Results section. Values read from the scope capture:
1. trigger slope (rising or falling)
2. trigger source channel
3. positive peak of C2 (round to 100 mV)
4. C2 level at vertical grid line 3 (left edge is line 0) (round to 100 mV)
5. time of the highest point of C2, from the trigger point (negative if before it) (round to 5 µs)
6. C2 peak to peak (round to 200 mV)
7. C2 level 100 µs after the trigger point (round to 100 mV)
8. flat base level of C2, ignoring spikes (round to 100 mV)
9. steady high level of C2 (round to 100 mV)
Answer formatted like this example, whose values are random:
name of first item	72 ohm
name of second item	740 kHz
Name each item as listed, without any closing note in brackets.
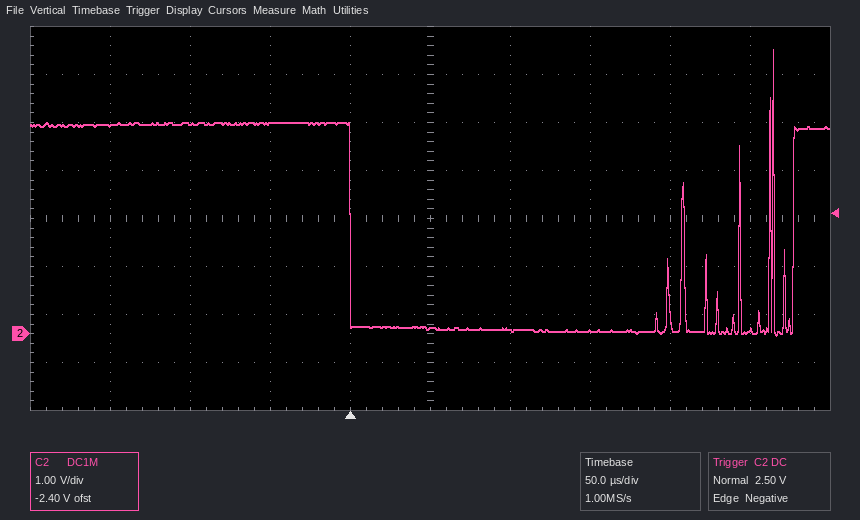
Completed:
trigger slope	falling
trigger source channel	C2
positive peak of C2	5.9 V
C2 level at vertical grid line 3 (left edge is line 0)	4.4 V
time of the highest point of C2, from the trigger point (negative if before it)	+265 µs
C2 peak to peak	6.0 V
C2 level 100 µs after the trigger point	100 mV
flat base level of C2, ignoring spikes	100 mV
steady high level of C2	4.4 V
